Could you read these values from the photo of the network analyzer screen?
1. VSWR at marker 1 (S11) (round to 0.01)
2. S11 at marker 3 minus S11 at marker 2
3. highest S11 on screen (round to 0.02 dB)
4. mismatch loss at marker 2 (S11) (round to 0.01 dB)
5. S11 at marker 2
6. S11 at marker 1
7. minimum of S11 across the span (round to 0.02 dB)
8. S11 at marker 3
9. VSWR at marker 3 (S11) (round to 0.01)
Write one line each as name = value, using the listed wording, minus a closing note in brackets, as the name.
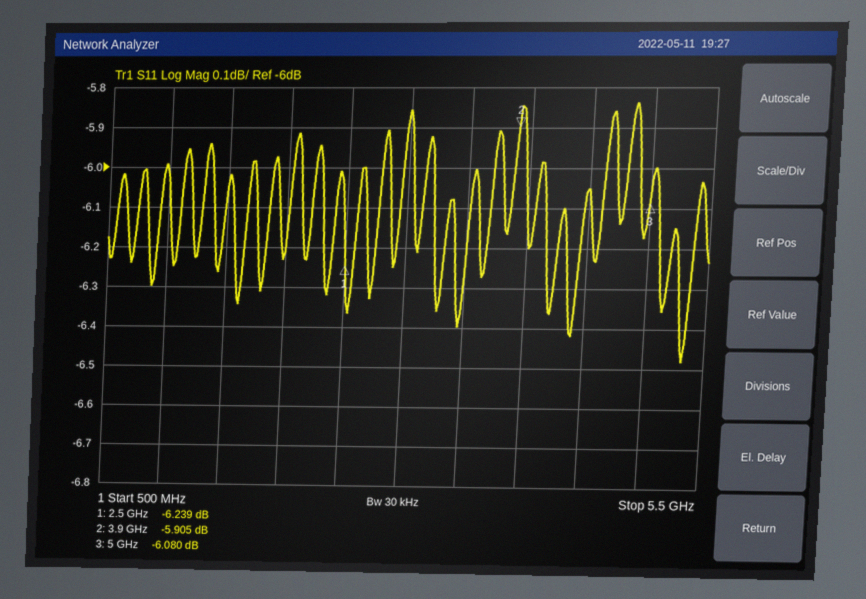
VSWR at marker 1 (S11) = 2.90
S11 at marker 3 minus S11 at marker 2 = -0.175 dB
highest S11 on screen = -5.84 dB
mismatch loss at marker 2 (S11) = 1.29 dB
S11 at marker 2 = -5.905 dB
S11 at marker 1 = -6.239 dB
minimum of S11 across the span = -6.48 dB
S11 at marker 3 = -6.080 dB
VSWR at marker 3 (S11) = 2.97
